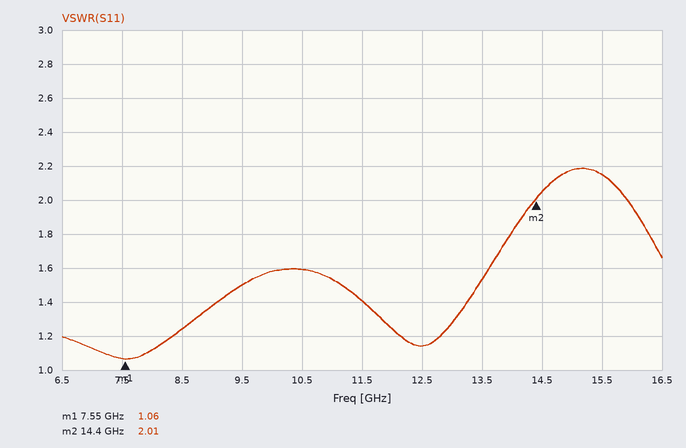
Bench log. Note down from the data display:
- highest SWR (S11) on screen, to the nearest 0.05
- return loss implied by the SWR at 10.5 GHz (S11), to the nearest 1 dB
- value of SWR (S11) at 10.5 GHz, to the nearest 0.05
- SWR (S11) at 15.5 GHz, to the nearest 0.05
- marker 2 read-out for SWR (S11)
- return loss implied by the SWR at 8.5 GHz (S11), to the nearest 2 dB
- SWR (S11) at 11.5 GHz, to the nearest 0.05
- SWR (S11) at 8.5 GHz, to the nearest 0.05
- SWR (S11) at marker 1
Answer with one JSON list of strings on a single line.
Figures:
["2.20", "13 dB", "1.60", "2.15", "2.01", "20 dB", "1.40", "1.25", "1.06"]
